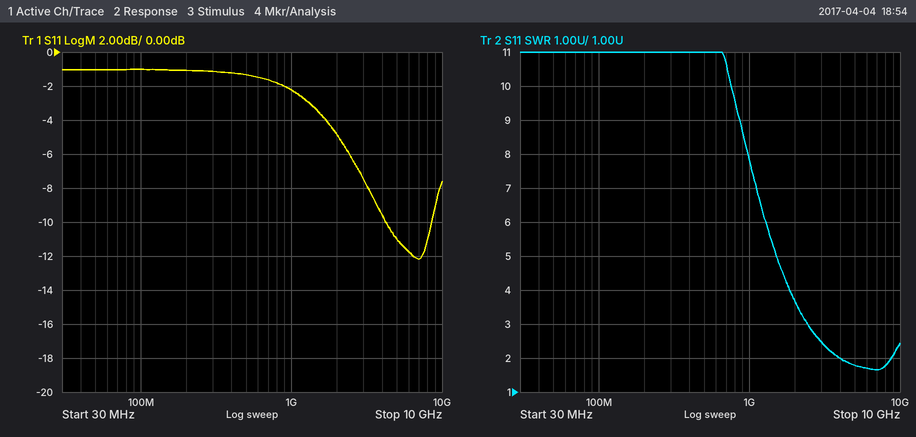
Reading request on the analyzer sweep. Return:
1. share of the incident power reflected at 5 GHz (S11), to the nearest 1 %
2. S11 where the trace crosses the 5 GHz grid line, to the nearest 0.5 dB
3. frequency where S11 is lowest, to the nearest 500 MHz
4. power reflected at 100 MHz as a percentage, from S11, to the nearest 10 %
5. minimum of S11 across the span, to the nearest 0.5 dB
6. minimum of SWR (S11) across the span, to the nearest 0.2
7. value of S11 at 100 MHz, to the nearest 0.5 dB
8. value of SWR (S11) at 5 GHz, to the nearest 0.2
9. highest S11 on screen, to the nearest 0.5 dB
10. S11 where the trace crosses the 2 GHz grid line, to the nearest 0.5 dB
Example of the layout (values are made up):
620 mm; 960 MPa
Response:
8 %; -11.0 dB; 7.0 GHz; 80 %; -12.0 dB; 1.6; -1.0 dB; 1.8; -1.0 dB; -5.0 dB
